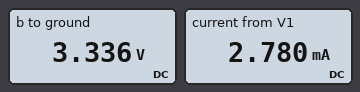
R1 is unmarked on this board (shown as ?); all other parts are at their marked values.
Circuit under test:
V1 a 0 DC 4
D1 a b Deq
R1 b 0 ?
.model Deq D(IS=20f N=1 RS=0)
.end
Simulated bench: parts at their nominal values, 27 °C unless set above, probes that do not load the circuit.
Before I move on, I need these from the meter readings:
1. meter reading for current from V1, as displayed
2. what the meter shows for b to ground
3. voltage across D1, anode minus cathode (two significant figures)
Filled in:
2.780 mA
3.336 V
660 mV
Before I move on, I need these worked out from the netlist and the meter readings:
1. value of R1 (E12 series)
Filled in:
1.2 kΩ
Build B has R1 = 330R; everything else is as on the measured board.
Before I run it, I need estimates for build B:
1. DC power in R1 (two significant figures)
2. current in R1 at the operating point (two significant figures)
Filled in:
33 mW
10 mA
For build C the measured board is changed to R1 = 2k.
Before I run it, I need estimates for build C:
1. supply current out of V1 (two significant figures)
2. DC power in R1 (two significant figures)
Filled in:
1.7 mA
5.6 mW
